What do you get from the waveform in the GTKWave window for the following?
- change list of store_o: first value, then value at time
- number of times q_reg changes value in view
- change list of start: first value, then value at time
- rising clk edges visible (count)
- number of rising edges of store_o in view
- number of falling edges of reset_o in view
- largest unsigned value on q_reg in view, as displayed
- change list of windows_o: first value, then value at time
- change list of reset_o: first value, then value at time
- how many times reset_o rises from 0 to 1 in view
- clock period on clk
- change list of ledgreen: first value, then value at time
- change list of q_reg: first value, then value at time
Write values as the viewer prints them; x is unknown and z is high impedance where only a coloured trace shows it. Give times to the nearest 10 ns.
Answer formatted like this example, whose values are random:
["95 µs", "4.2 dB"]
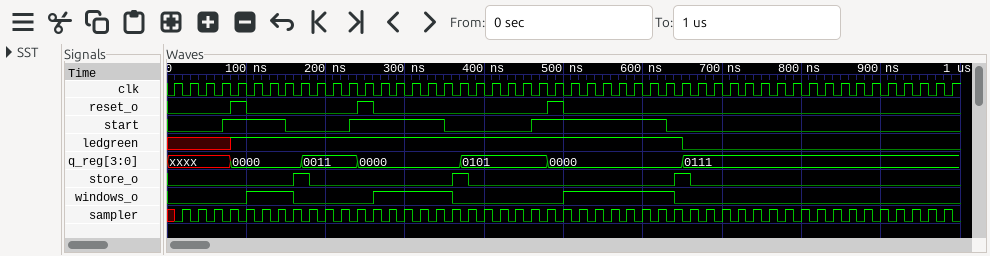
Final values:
["0, 1 at 160 ns, 0 at 180 ns, 1 at 360 ns, 0 at 380 ns, 1 at 640 ns, 0 at 660 ns", "6", "0, 1 at 70 ns, 0 at 150 ns, 1 at 230 ns, 0 at 350 ns, 1 at 460 ns, 0 at 630 ns", "50", "3", "3", "0111", "0, 1 at 100 ns, 0 at 160 ns, 1 at 260 ns, 0 at 360 ns, 1 at 500 ns, 0 at 640 ns", "0, 1 at 80 ns, 0 at 100 ns, 1 at 240 ns, 0 at 260 ns, 1 at 480 ns, 0 at 500 ns", "3", "20 ns", "x, 1 at 80 ns, 0 at 650 ns", "xxxx, 0000 at 80 ns, 0011 at 170 ns, 0000 at 240 ns, 0101 at 370 ns, 0000 at 480 ns, 0111 at 650 ns"]
